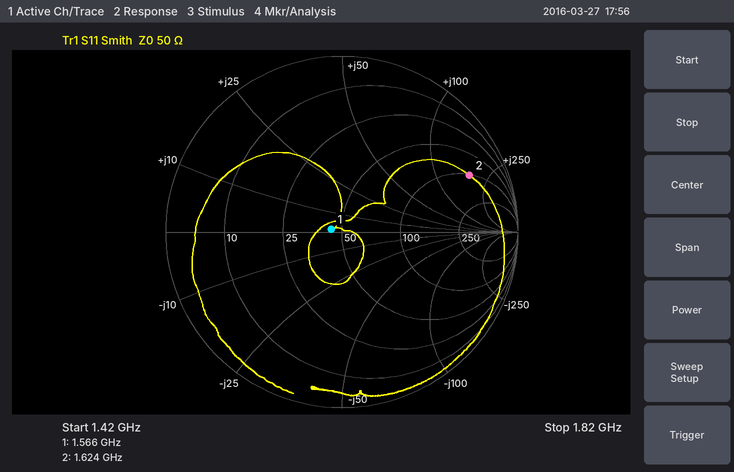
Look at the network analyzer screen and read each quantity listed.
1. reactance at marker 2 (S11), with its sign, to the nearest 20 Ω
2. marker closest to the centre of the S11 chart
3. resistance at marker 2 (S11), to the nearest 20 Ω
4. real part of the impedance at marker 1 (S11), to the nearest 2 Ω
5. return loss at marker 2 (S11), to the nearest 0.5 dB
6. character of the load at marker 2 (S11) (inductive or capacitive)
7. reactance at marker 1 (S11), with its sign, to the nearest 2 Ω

+180 Ω
marker 1
100 Ω
44 Ω
2.0 dB
inductive
+2 Ω
